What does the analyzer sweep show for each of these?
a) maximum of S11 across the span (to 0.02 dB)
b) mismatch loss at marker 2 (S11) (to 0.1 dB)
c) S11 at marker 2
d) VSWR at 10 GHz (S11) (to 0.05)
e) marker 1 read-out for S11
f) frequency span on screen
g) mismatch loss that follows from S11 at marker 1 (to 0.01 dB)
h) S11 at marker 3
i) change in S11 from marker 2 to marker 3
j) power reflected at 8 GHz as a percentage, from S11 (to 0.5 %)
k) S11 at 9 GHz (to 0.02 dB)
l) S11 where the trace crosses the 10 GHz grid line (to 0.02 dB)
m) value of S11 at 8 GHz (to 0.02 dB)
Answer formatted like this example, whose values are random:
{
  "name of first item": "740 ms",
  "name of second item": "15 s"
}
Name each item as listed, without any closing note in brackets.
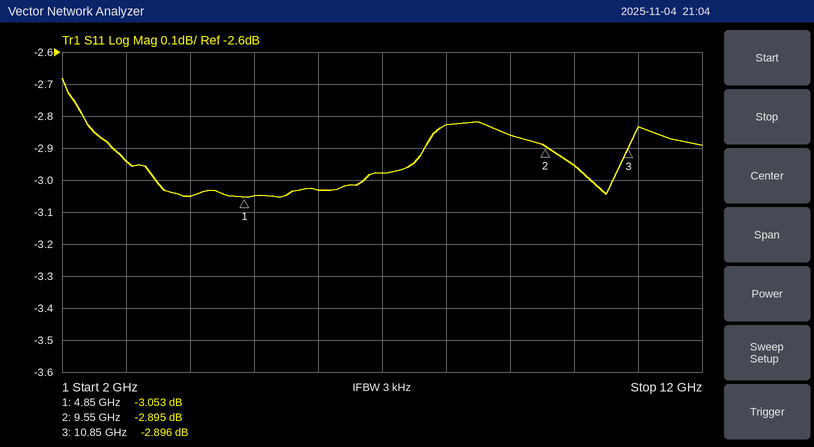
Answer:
{
  "maximum of S11 across the span": "-2.68 dB",
  "mismatch loss at marker 2 (S11)": "3.1 dB",
  "S11 at marker 2": "-2.895 dB",
  "VSWR at 10 GHz (S11)": "5.95",
  "marker 1 read-out for S11": "-3.053 dB",
  "frequency span on screen": "10 GHz",
  "mismatch loss that follows from S11 at marker 1": "2.97 dB",
  "S11 at marker 3": "-2.896 dB",
  "change in S11 from marker 2 to marker 3": "-0.001 dB",
  "power reflected at 8 GHz as a percentage, from S11": "52.0 %",
  "S11 at 9 GHz": "-2.86 dB",
  "S11 where the trace crosses the 10 GHz grid line": "-2.96 dB",
  "value of S11 at 8 GHz": "-2.82 dB"
}
